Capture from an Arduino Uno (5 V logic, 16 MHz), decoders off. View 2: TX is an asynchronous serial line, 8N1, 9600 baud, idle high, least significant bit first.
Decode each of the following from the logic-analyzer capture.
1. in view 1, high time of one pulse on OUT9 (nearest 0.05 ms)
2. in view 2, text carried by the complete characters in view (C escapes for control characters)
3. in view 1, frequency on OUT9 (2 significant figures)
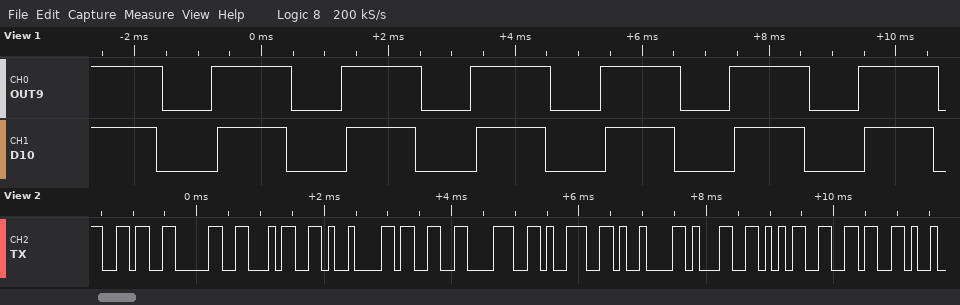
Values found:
1.25 ms
"604\t389\t156"
490 Hz
